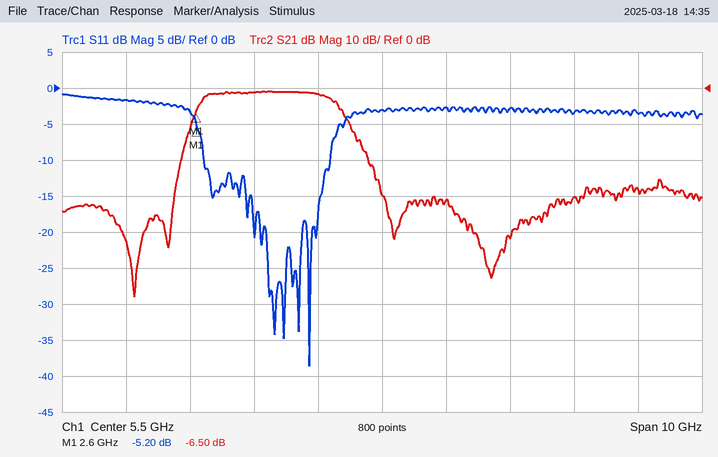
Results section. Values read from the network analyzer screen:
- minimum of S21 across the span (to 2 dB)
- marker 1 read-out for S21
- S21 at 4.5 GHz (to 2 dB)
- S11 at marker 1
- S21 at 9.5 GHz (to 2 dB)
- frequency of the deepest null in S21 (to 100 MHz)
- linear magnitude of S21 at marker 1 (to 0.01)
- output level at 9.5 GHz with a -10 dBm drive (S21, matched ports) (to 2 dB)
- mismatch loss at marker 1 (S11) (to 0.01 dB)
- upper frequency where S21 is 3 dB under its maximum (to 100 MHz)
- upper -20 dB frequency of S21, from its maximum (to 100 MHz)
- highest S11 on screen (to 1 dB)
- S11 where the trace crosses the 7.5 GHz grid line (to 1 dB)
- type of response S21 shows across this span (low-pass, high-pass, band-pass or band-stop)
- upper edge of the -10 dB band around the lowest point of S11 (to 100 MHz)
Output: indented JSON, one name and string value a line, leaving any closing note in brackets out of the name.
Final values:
{
  "minimum of S21 across the span": "-58 dB",
  "marker 1 read-out for S21": "-6.50 dB",
  "S21 at 4.5 GHz": "-2 dB",
  "S11 at marker 1": "-5.20 dB",
  "S21 at 9.5 GHz": "-28 dB",
  "frequency of the deepest null in S21": "1.6 GHz",
  "linear magnitude of S21 at marker 1": "0.47",
  "output level at 9.5 GHz with a -10 dBm drive (S21, matched ports)": "-38 dBm",
  "mismatch loss at marker 1 (S11)": "1.56 dB",
  "upper frequency where S21 is 3 dB under its maximum": "4.8 GHz",
  "upper -20 dB frequency of S21, from its maximum": "5.3 GHz",
  "highest S11 on screen": "-1 dB",
  "S11 where the trace crosses the 7.5 GHz grid line": "-3 dB",
  "type of response S21 shows across this span": "band-pass",
  "upper edge of the -10 dB band around the lowest point of S11": "4.7 GHz"
}
